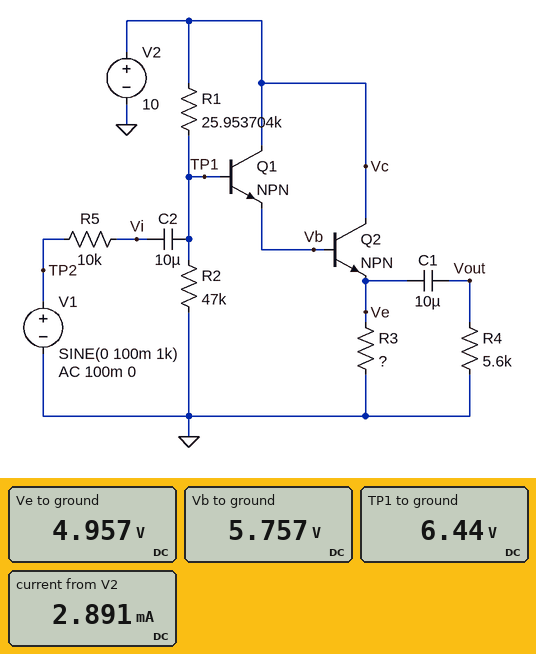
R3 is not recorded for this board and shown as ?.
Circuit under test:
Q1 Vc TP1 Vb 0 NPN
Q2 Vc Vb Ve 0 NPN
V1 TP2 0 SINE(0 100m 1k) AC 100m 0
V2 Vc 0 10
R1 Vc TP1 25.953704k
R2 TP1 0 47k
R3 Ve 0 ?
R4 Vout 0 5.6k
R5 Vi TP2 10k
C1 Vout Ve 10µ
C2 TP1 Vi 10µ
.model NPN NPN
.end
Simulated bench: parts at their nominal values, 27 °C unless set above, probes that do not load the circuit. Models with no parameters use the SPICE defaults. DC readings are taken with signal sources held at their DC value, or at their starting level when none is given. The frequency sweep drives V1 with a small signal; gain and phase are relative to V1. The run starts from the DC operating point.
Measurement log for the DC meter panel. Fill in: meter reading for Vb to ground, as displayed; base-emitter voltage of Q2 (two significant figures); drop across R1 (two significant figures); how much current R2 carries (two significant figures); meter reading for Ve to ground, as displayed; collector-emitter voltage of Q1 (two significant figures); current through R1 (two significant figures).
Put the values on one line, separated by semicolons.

5.757 V; 800 mV; 3.6 V; 140 µA; 4.957 V; 4.2 V; 140 µA
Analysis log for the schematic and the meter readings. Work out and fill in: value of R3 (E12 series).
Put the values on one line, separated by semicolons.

1.8 kΩ
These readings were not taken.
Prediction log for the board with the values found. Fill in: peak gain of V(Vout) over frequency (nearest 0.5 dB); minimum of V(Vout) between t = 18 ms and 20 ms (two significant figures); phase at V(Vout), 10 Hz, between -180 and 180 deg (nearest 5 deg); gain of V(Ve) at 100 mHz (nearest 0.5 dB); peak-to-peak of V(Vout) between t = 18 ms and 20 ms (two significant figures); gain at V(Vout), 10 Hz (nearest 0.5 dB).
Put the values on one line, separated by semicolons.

-4.0 dB; -62 mV; 20 deg; -20.0 dB; 120 mV; -4.5 dB
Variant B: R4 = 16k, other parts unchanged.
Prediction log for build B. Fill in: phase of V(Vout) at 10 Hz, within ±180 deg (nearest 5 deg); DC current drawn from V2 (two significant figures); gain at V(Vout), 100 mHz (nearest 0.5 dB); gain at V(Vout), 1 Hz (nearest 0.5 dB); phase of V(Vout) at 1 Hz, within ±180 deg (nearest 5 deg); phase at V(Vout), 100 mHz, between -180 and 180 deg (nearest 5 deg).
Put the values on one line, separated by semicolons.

10 deg; 2.9 mA; -40.0 dB; -8.5 dB; 75 deg; 165 deg
